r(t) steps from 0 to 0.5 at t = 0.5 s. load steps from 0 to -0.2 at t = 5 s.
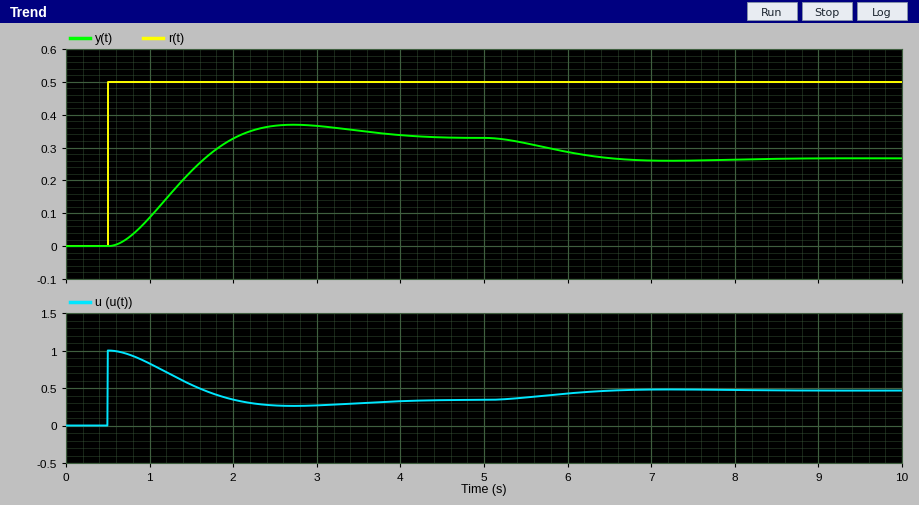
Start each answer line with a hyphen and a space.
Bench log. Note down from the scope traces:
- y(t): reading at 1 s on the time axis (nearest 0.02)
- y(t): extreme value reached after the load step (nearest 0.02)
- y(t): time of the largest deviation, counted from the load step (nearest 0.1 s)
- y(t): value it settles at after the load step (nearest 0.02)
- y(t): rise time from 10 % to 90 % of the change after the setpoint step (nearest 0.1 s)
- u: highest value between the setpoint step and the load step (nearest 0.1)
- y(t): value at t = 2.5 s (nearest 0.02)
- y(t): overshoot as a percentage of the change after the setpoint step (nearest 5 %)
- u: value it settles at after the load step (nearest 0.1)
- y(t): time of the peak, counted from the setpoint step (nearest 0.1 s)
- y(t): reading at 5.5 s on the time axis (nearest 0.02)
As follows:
- 0.08
- 0.26
- 2.2 s
- 0.26
- 1.0 s
- 1.0
- 0.36
- 10 %
- 0.5
- 2.2 s
- 0.32
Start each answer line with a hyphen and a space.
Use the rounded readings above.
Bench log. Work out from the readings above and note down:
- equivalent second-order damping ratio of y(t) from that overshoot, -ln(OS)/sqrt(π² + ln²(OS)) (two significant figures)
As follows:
- 0.59
